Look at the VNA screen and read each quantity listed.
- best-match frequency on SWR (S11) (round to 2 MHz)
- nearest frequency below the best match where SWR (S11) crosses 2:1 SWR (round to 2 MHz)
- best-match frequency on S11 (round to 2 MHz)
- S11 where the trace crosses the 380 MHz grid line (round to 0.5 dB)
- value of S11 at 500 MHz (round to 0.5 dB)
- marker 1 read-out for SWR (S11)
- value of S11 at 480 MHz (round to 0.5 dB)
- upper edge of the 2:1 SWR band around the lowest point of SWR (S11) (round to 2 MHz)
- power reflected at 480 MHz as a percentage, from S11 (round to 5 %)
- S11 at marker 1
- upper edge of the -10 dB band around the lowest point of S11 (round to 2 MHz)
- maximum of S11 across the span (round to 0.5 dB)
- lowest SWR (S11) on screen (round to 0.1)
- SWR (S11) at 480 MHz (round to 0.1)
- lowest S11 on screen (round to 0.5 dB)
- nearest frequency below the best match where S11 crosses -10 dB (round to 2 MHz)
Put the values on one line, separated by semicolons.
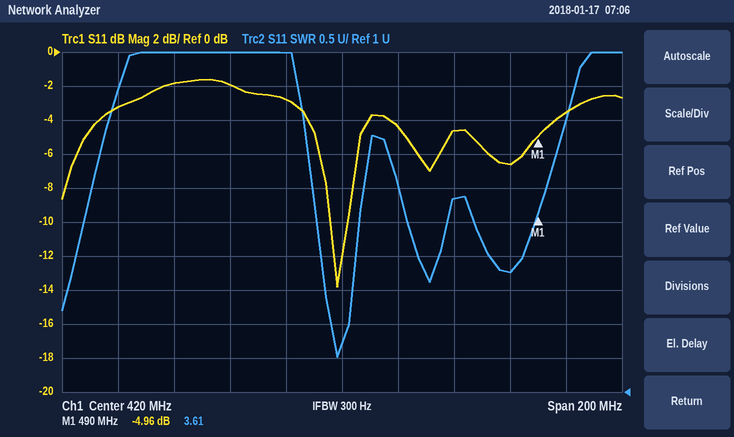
418 MHz; 416 MHz; 418 MHz; -2.0 dB; -3.5 dB; 3.61; -6.5 dB; 422 MHz; 20 %; -4.96 dB; 422 MHz; -1.5 dB; 1.5; 2.8; -14.0 dB; 416 MHz
